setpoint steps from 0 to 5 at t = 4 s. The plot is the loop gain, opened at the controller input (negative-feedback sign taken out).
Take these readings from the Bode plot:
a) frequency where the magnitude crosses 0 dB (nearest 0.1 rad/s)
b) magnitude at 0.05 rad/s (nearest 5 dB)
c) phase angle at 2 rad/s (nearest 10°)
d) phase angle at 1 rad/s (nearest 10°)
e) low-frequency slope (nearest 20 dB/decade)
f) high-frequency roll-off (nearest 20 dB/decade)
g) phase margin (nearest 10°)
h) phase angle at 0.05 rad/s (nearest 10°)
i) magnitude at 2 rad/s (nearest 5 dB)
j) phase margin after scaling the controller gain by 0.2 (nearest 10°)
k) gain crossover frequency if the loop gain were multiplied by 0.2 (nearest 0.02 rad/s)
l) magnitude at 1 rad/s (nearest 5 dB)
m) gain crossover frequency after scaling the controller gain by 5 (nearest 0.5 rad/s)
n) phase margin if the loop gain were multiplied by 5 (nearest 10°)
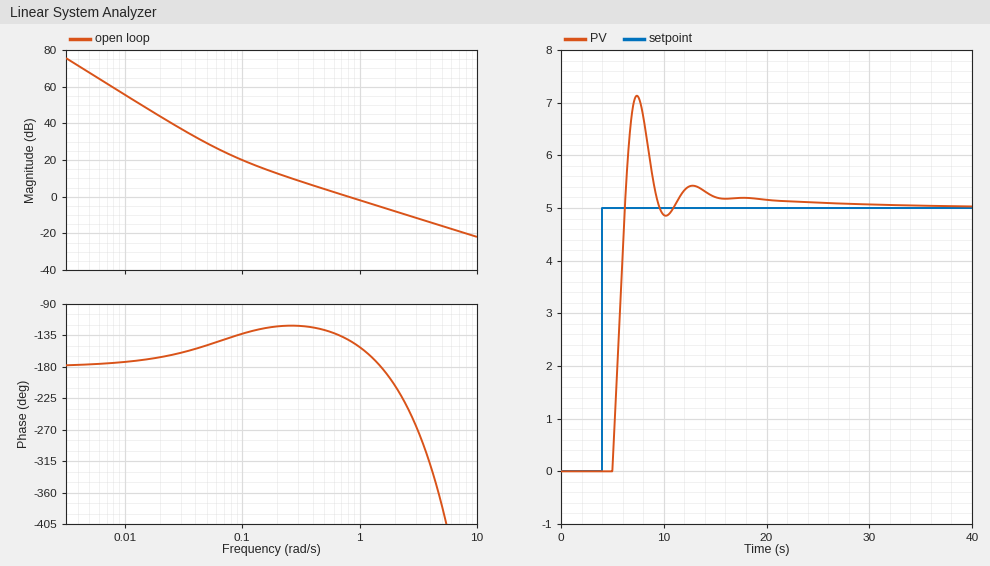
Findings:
0.8 rad/s
30 dB
-210°
-150°
-40 dB/decade
-20 dB/decade
40°
-150°
-10 dB
60°
0.18 rad/s
0 dB
4.0 rad/s
-140°
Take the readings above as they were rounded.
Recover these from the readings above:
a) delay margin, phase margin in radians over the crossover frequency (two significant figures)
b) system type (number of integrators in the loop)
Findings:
0.87 s
2
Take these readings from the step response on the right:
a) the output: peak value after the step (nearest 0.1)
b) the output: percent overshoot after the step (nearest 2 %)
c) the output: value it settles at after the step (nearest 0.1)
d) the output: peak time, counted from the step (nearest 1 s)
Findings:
7.1
42 %
5.0
3 s
